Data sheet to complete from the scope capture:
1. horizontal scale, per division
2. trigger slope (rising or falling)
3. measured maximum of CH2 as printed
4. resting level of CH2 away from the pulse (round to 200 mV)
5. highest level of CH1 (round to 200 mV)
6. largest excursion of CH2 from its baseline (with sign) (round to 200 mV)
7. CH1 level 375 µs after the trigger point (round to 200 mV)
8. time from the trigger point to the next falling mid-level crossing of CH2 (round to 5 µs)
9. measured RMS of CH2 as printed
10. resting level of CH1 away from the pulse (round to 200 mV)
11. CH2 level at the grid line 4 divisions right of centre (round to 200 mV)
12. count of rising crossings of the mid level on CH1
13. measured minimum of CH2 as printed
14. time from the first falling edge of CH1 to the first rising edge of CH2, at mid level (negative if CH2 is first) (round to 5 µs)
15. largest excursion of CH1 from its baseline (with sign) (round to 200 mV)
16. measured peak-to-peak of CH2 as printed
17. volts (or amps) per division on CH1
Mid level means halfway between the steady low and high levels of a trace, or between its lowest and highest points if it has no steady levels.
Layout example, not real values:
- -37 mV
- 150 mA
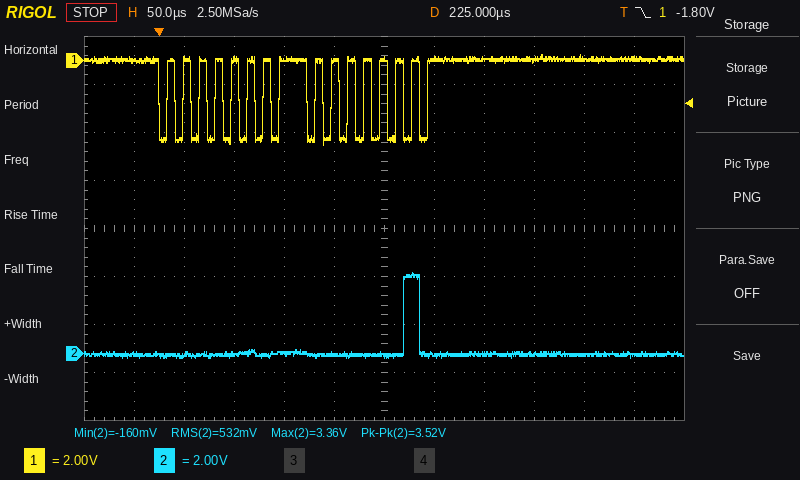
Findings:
- 50 µs
- falling
- 3.36 V
- 0.0 V
- 200 mV
- +3.4 V
- 0.0 V
- 260 µs
- 532 mV
- 0.0 V
- 0.0 V
- 16
- -160 mV
- +245 µs
- -3.6 V
- 3.52 V
- 2 V
